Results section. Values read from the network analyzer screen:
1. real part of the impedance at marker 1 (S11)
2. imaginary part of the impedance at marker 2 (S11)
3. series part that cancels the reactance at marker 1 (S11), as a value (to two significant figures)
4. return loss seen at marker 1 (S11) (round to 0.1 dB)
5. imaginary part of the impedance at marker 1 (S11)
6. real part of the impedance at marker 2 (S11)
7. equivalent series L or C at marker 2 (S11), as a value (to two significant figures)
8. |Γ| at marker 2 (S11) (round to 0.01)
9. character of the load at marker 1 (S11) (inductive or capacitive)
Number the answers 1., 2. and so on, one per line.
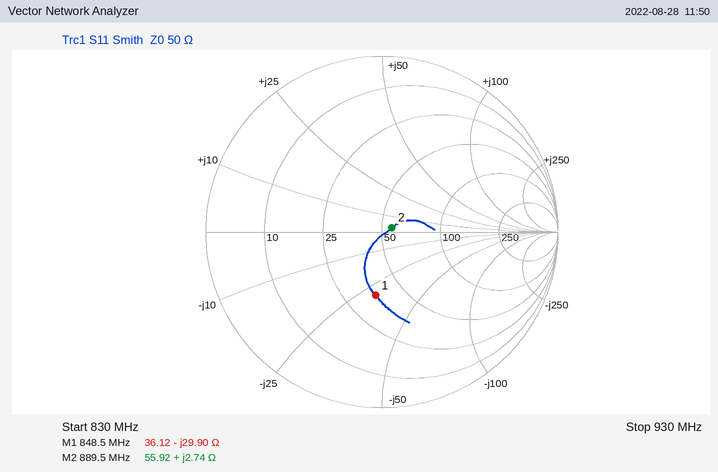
1. 36.12 Ω
2. +2.74 Ω
3. 5.6 nH
4. 8.8 dB
5. -29.90 Ω
6. 55.92 Ω
7. 490 pH
8. 0.06
9. capacitive
